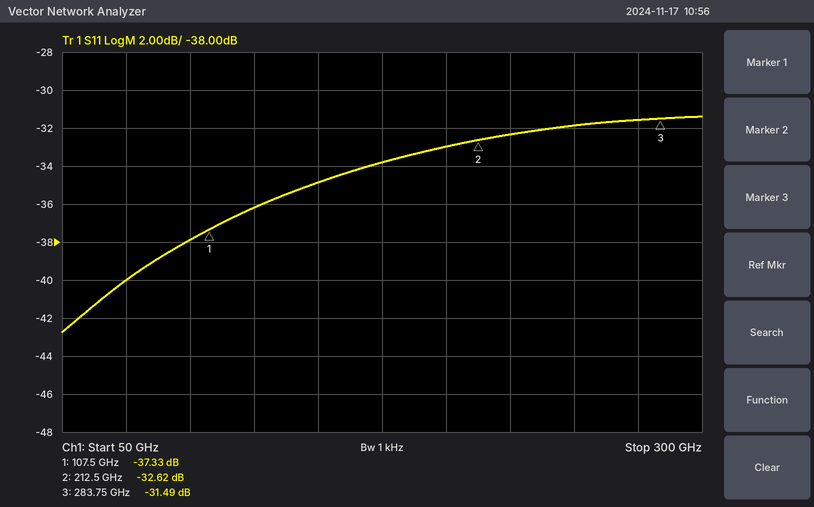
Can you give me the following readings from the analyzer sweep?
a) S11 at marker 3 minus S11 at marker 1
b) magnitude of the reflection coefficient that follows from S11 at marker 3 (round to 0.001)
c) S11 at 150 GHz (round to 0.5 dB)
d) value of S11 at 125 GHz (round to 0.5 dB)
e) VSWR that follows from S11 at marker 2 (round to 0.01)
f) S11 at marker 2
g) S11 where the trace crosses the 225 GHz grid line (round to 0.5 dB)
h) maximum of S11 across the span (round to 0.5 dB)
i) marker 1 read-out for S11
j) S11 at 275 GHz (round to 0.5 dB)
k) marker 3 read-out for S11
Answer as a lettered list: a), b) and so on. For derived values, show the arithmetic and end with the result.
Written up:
a) -31.49 − (-37.33) = 5.84 dB
b) 10^(-31.49/20) ≈ 0.027
c) -35.0 dB
d) -36.0 dB
e) (1 + 0.0234)/(1 − 0.0234) ≈ 1.05
f) -32.62 dB
g) -32.5 dB
h) -31.5 dB
i) -37.33 dB
j) -31.5 dB
k) -31.49 dB
